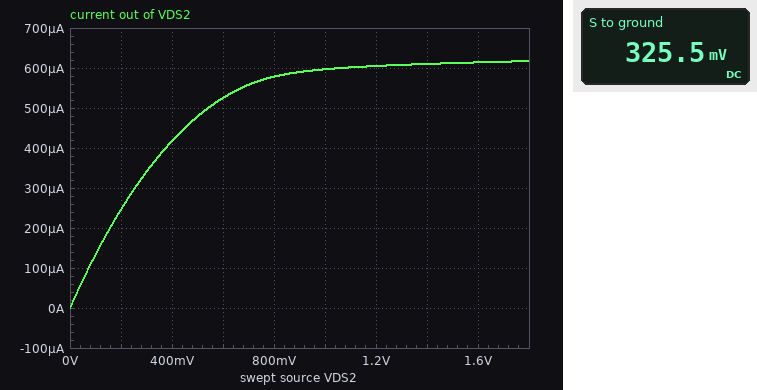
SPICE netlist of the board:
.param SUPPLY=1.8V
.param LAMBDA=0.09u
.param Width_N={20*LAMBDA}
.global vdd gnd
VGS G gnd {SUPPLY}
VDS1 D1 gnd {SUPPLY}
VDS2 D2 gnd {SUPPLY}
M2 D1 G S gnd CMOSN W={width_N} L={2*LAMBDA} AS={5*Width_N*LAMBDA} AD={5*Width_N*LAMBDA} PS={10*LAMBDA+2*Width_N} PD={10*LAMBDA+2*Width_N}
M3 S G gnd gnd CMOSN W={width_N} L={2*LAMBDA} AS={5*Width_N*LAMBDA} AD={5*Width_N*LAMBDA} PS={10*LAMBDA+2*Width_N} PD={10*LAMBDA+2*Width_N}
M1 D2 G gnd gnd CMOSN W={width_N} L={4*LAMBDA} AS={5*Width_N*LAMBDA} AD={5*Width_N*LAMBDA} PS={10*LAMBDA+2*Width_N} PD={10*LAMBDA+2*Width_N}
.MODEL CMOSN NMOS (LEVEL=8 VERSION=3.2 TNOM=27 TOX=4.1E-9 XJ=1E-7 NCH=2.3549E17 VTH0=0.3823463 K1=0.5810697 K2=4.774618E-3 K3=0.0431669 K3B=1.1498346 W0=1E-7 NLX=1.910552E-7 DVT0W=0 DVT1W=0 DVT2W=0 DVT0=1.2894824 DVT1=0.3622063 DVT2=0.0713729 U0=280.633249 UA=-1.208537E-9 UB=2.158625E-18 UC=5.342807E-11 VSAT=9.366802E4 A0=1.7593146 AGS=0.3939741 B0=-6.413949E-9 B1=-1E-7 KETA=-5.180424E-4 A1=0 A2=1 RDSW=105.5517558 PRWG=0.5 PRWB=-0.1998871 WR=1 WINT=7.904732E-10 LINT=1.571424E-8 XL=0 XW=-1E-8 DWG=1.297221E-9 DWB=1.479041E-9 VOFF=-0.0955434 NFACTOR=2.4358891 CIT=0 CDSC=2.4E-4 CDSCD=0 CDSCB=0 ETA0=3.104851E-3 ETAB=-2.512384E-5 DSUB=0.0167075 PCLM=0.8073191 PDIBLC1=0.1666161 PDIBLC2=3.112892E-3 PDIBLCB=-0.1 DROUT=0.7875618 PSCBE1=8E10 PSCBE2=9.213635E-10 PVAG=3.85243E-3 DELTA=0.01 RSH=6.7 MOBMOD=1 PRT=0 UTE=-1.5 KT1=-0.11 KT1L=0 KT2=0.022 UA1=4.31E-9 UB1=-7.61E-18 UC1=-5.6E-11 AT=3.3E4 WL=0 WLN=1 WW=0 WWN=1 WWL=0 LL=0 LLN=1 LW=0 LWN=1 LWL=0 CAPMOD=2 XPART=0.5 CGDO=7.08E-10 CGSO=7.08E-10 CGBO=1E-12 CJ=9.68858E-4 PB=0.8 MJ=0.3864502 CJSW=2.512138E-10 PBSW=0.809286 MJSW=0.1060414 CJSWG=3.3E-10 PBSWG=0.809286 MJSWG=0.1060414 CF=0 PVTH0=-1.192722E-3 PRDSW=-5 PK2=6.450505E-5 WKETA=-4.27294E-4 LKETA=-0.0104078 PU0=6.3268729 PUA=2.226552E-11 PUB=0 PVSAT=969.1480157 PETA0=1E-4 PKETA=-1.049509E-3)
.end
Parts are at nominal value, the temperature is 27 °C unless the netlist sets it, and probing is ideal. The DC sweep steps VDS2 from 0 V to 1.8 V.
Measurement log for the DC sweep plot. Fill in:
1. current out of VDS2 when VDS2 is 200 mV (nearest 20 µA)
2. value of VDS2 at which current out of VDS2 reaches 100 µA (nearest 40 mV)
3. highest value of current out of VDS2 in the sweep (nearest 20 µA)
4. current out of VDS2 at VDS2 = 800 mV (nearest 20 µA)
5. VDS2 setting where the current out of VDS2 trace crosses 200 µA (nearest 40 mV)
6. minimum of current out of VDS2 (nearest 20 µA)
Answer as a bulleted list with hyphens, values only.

- 240 µA
- 80 mV
- 620 µA
- 580 µA
- 160 mV
- 0 A
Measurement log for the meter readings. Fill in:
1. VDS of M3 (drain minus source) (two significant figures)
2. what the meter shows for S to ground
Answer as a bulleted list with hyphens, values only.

- 330 mV
- 325.5 mV
